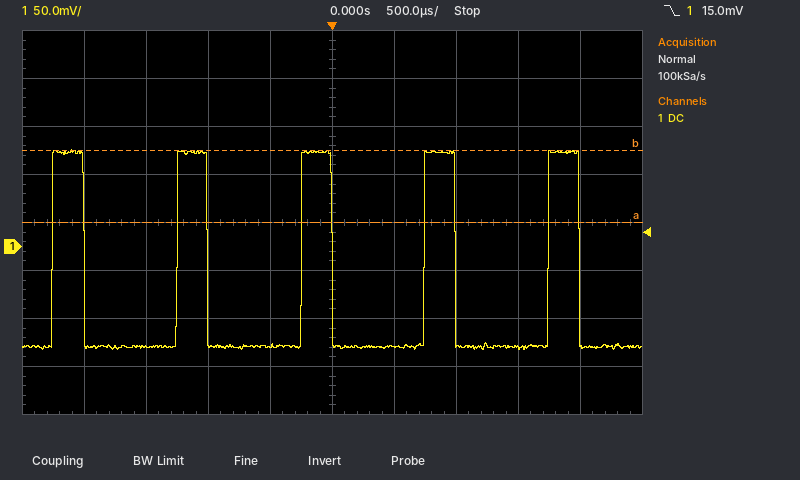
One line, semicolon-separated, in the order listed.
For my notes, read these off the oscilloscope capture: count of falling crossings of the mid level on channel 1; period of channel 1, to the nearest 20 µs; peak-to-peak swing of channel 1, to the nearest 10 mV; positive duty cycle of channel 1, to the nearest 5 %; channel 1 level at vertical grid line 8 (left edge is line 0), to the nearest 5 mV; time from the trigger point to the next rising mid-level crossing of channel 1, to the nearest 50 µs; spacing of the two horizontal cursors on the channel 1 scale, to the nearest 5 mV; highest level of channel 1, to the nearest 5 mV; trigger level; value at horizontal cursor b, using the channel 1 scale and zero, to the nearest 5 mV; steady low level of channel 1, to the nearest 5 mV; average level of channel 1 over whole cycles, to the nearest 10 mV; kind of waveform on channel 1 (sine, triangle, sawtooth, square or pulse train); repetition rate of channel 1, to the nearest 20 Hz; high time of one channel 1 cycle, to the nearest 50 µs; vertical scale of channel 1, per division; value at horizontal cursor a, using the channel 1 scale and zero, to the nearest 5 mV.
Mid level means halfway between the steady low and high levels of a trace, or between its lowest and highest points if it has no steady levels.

5; 1.00 ms; 210 mV; 25 %; -105 mV; 750 µs; 75 mV; 100 mV; 15.0 mV; 100 mV; -105 mV; -50 mV; pulse train; 1.00 kHz; 250 µs; 50 mV; 25 mV
